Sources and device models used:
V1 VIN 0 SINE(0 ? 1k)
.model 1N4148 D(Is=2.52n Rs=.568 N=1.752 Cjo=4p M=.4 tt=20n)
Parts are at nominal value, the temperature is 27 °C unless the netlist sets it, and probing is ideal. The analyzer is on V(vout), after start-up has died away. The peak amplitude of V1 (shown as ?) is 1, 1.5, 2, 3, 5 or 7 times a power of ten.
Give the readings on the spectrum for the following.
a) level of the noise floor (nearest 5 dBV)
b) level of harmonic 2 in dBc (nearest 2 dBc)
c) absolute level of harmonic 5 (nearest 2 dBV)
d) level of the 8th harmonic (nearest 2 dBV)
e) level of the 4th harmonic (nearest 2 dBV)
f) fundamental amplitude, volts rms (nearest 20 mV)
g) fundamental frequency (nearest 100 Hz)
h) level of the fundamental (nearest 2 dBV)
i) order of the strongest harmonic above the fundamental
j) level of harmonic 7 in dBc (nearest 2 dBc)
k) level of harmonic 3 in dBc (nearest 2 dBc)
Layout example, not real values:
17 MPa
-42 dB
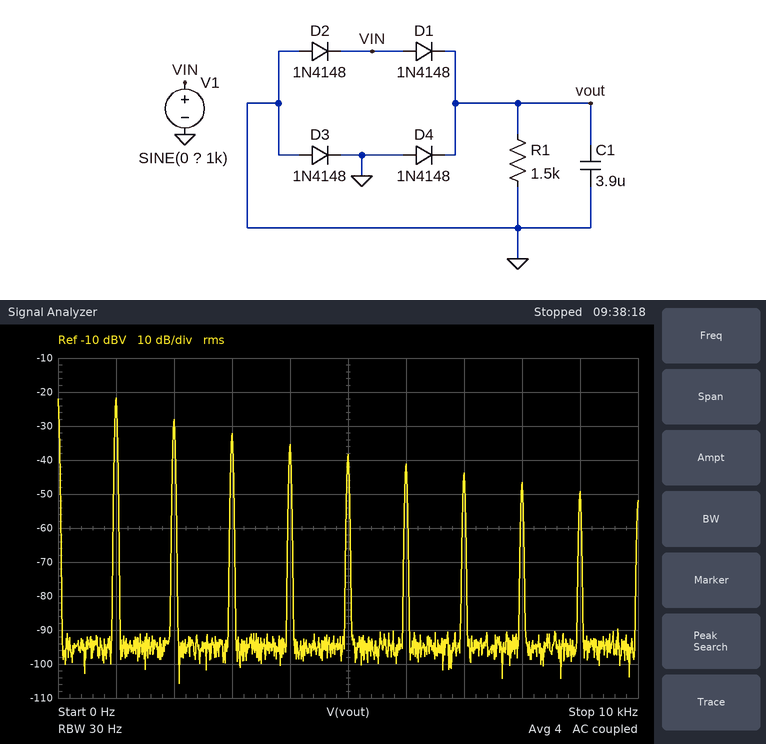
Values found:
-95 dBV
-6 dBc
-38 dBV
-46 dBV
-36 dBV
80 mV
1.0 kHz
-22 dBV
2
-22 dBc
-10 dBc
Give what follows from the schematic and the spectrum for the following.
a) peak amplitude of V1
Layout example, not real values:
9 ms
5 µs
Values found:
3 V
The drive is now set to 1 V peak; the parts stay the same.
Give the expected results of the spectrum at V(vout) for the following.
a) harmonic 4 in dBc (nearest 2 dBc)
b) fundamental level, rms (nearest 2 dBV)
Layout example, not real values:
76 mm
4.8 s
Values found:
-16 dBc
-38 dBV
